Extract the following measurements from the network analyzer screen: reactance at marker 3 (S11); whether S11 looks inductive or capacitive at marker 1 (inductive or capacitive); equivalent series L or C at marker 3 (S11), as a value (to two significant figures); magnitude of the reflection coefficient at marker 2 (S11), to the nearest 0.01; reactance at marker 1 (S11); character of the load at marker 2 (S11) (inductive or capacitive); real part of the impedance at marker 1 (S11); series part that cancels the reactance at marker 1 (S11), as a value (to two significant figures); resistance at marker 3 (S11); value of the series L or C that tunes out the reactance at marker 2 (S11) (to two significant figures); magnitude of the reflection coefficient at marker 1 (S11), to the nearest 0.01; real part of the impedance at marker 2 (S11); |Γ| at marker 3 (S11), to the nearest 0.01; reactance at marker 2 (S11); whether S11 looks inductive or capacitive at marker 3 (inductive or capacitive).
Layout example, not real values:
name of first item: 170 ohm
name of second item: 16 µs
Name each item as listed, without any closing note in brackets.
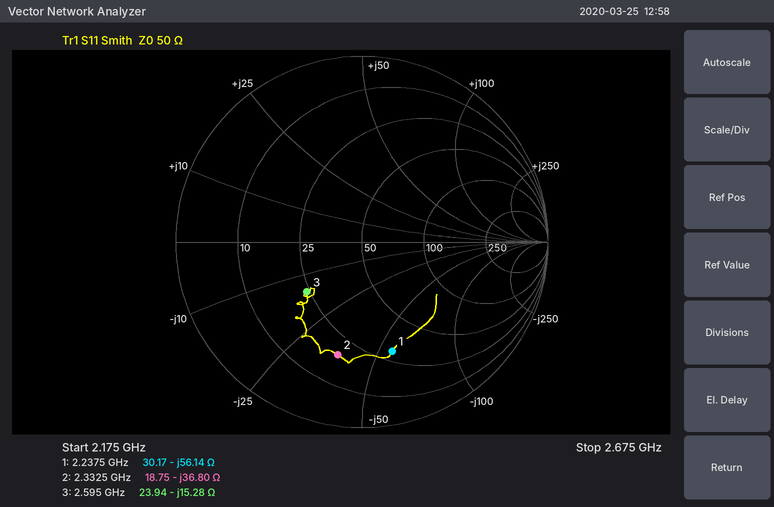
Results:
reactance at marker 3: -15.28 Ω
whether S11 looks inductive or capacitive at marker 1: capacitive
equivalent series L or C at marker 3 (S11), as a value: 4.0 pF
magnitude of the reflection coefficient at marker 2 (S11), to the nearest 0.01: 0.62
reactance at marker 1: -56.14 Ω
character of the load at marker 2 (S11): capacitive
real part of the impedance at marker 1: 30.17 Ω
series part that cancels the reactance at marker 1 (S11), as a value: 4.0 nH
resistance at marker 3: 23.94 Ω
value of the series L or C that tunes out the reactance at marker 2 (S11): 2.5 nH
magnitude of the reflection coefficient at marker 1 (S11), to the nearest 0.01: 0.61
real part of the impedance at marker 2: 18.75 Ω
|Γ| at marker 3 (S11), to the nearest 0.01: 0.40
reactance at marker 2: -36.80 Ω
whether S11 looks inductive or capacitive at marker 3: capacitive
